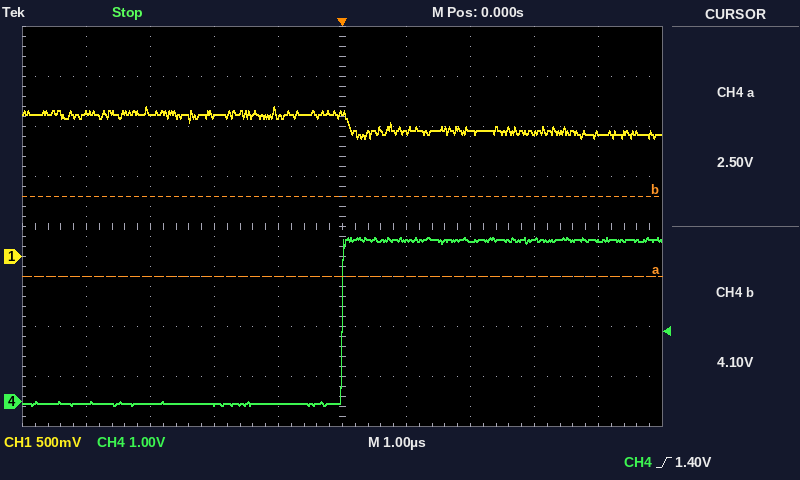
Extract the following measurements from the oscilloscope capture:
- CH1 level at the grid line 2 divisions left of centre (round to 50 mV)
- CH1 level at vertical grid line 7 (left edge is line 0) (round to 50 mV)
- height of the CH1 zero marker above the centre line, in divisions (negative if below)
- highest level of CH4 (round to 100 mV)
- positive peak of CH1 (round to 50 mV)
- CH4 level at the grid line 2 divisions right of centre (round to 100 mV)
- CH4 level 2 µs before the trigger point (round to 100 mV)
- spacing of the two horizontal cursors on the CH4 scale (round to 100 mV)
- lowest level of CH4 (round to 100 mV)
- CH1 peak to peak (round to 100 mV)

1.40 V
1.25 V
-0.6 div
3.3 V
1.50 V
3.2 V
-100 mV
1.6 V
-100 mV
300 mV
